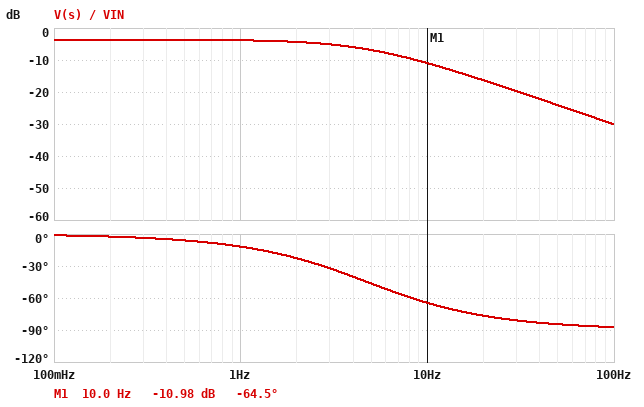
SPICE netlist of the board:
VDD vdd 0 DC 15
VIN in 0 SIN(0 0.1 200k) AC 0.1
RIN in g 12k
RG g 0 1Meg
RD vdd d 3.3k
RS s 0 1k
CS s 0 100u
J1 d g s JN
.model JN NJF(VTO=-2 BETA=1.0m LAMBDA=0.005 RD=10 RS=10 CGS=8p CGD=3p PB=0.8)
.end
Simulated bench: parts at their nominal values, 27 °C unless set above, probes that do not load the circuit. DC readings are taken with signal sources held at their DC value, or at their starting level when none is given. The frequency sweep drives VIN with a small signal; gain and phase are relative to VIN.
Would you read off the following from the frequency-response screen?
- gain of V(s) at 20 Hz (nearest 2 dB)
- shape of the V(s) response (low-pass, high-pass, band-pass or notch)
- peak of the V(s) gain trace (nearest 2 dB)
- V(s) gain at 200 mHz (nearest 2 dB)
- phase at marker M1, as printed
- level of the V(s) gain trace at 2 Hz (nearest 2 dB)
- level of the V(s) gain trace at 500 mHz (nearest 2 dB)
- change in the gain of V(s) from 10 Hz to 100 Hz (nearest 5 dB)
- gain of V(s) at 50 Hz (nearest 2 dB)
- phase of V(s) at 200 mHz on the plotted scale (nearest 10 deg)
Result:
-16 dB
low-pass
-4 dB
-4 dB
-64.5 deg
-4 dB
-4 dB
-20 dB
-24 dB
0 deg
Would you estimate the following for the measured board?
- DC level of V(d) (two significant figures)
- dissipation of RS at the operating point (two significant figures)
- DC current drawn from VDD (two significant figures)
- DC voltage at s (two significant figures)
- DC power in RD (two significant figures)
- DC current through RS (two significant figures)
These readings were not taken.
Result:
12 V
1.0 mW
1.0 mA
1.0 V
3.4 mW
1.0 mA
